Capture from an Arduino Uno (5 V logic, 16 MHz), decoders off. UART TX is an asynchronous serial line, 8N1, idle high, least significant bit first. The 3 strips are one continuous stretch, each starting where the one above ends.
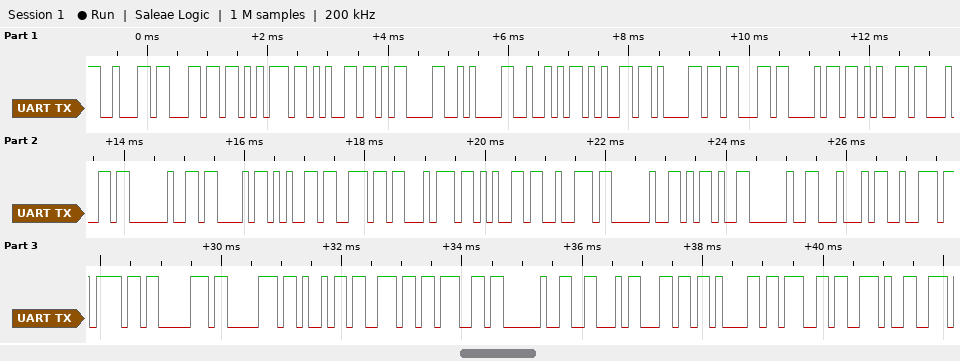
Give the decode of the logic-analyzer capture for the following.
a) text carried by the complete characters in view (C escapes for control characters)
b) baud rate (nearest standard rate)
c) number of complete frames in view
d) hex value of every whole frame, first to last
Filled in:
"blue\r\nReached Center - Dropping Flag."
9600 baud
37
0x62 0x6C 0x75 0x65 0x0D 0x0A 0x52 0x65 0x61 0x63 0x68 0x65 0x64 0x20 0x43 0x65 0x6E 0x74 0x65 0x72 0x20 0x2D 0x20 0x44 0x72 0x6F 0x70 0x70 0x69 0x6E 0x67 0x20 0x46 0x6C 0x61 0x67 0x2E
